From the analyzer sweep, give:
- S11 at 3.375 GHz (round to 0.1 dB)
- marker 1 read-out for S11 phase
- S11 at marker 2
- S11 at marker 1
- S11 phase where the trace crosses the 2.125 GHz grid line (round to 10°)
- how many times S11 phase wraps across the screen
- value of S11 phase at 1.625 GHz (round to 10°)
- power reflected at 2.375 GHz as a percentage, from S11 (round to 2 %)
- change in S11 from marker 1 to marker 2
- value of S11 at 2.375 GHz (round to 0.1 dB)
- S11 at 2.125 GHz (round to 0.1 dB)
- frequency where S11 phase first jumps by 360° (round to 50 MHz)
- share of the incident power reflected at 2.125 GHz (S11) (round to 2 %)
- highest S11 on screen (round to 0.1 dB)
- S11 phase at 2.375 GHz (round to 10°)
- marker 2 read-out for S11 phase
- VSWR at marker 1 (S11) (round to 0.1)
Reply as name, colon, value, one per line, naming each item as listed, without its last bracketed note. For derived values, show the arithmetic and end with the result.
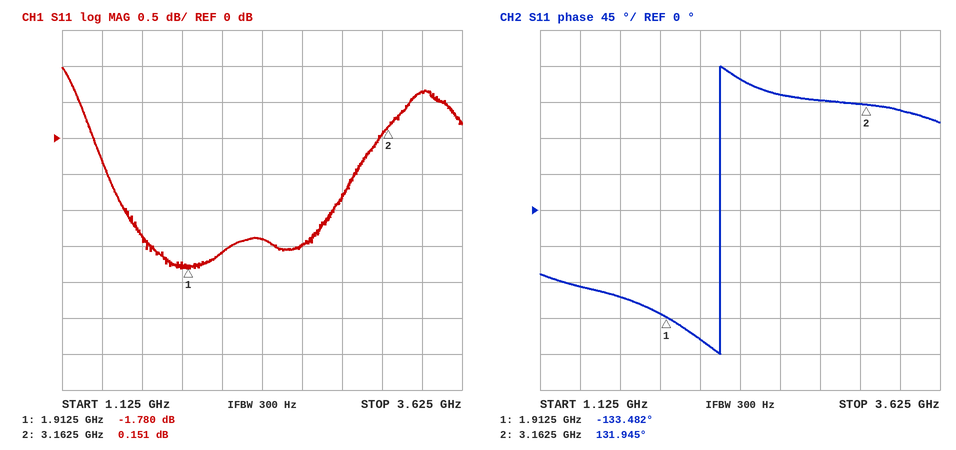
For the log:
S11 at 3.375 GHz: 0.6 dB
marker 1 read-out for S11 phase: -133.482°
S11 at marker 2: 0.151 dB
S11 at marker 1: -1.780 dB
S11 phase where the trace crosses the 2.125 GHz grid line: -160°
how many times S11 phase wraps across the screen: 1
value of S11 phase at 1.625 GHz: -110°
power reflected at 2.375 GHz as a percentage, from S11: 10^(-1.4/10) ≈ 72 %
change in S11 from marker 1 to marker 2: 0.151 − (-1.78) = 1.931 dB
value of S11 at 2.375 GHz: -1.4 dB
S11 at 2.125 GHz: -1.6 dB
frequency where S11 phase first jumps by 360°: 2.25 GHz
share of the incident power reflected at 2.125 GHz (S11): 10^(-1.6/10) ≈ 69.2 %, so 70 % to the nearest 2 %
highest S11 on screen: 1.0 dB
S11 phase at 2.375 GHz: 160°
marker 2 read-out for S11 phase: 131.945°
VSWR at marker 1 (S11): (1 + 0.8147)/(1 − 0.8147) ≈ 9.8
